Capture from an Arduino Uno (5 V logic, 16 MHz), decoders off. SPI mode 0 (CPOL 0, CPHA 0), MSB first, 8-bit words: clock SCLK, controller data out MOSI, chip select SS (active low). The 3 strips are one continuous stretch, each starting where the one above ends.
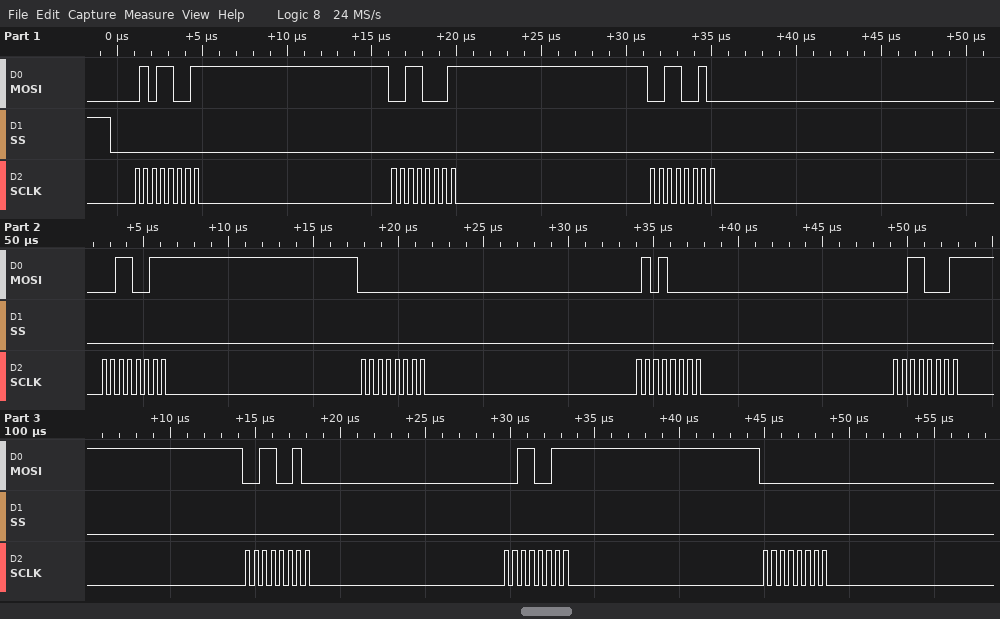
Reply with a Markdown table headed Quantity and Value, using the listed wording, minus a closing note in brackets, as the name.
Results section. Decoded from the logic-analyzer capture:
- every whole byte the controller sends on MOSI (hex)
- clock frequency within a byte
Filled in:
| Quantity | Value |
|---|---|
| every whole byte the controller sends on MOSI | 0x59 0x31 0x32 0x33 0x00 0x50 0x31 0x32 0x33 0x00 |
| clock frequency within a byte | 2 MHz |
